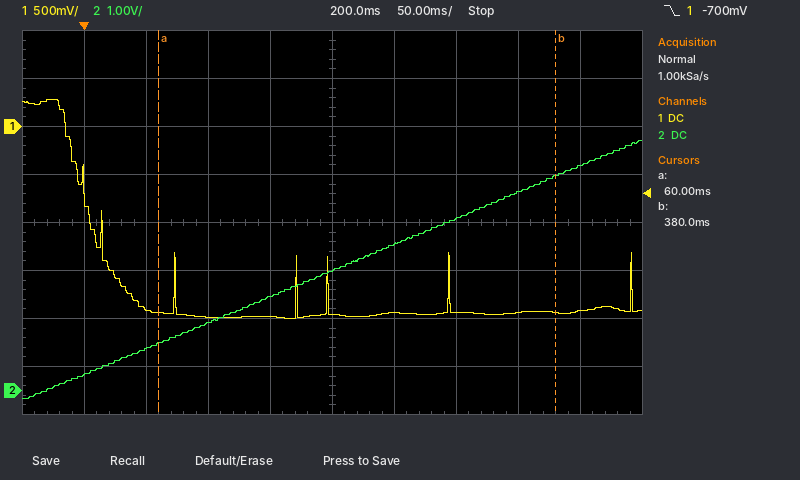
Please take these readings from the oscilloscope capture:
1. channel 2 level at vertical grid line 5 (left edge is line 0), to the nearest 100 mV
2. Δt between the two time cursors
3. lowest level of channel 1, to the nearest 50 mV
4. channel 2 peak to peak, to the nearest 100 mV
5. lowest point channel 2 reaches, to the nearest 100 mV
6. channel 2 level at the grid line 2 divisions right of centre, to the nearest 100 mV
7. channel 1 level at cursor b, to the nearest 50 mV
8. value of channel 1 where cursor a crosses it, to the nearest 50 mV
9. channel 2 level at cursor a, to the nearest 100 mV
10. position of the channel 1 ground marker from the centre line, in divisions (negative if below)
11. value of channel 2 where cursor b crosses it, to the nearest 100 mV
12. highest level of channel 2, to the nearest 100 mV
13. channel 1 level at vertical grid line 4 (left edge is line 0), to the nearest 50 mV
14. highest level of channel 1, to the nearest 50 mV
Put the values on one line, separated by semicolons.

2.5 V; 320 ms; -2.00 V; 5.4 V; -200 mV; 3.6 V; -1.95 V; -1.95 V; 1.0 V; +2.0 div; 4.5 V; 5.2 V; -2.00 V; 300 mV
